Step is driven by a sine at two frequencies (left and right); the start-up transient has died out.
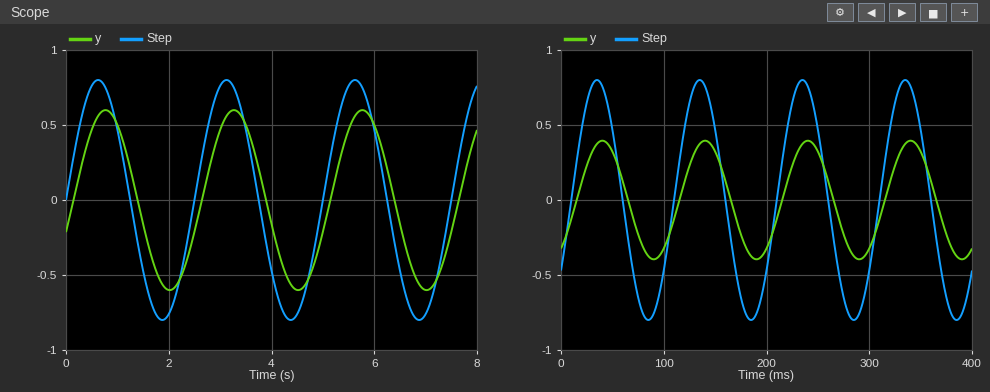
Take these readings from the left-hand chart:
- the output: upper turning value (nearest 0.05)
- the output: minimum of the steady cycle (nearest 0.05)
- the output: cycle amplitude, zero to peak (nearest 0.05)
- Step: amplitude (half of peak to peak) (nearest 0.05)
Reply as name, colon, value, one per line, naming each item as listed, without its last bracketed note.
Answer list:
the output: upper turning value: 0.60
the output: minimum of the steady cycle: -0.60
the output: cycle amplitude, zero to peak: 0.60
Step: amplitude (half of peak to peak): 0.80
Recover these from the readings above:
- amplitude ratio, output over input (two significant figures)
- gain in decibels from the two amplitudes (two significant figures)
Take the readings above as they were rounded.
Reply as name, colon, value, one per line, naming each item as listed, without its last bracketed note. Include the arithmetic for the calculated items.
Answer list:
amplitude ratio, output over input: 0.6 / 0.8 = 0.75
gain in decibels from the two amplitudes: 20 log10(0.6 / 0.8) = -2.5 dB
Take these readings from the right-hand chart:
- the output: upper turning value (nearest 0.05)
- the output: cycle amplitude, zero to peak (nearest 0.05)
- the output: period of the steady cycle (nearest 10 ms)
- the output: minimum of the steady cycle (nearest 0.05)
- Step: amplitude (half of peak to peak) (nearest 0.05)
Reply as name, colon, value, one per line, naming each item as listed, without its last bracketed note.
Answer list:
the output: upper turning value: 0.40
the output: cycle amplitude, zero to peak: 0.40
the output: period of the steady cycle: 100 ms
the output: minimum of the steady cycle: -0.40
Step: amplitude (half of peak to peak): 0.80
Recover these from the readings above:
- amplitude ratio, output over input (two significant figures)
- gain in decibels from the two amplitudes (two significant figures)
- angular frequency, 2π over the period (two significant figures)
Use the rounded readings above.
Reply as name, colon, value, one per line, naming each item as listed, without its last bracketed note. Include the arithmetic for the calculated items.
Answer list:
amplitude ratio, output over input: 0.4 / 0.8 = 0.50
gain in decibels from the two amplitudes: 20 log10(0.4 / 0.8) = -6.0 dB
angular frequency, 2π over the period: 2π / 100 = 0.063 rad/ms
